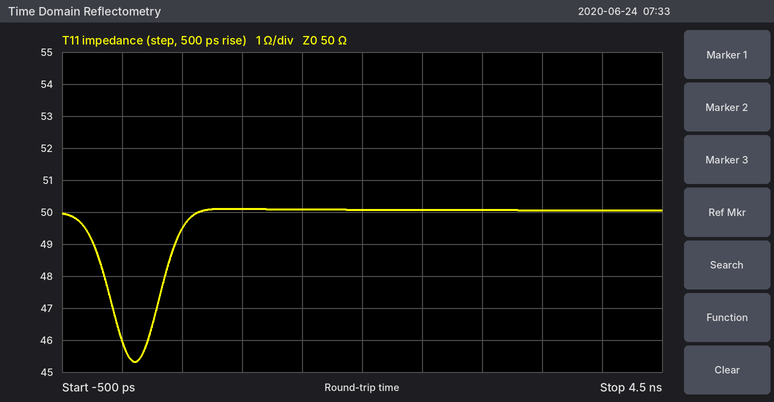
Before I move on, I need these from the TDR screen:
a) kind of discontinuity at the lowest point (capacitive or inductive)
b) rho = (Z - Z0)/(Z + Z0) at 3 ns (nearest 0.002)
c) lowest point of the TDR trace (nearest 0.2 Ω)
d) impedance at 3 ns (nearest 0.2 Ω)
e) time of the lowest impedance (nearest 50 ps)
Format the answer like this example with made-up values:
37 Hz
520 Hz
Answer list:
capacitive
0.000
45.4 Ω
50.0 Ω
100 ps
